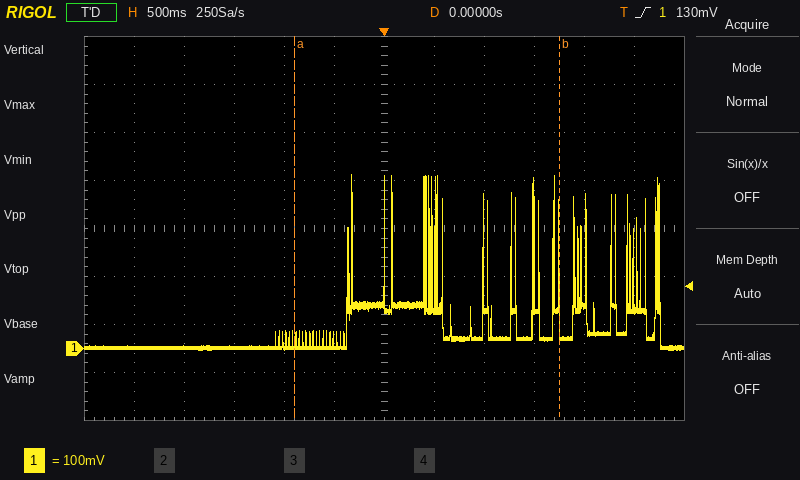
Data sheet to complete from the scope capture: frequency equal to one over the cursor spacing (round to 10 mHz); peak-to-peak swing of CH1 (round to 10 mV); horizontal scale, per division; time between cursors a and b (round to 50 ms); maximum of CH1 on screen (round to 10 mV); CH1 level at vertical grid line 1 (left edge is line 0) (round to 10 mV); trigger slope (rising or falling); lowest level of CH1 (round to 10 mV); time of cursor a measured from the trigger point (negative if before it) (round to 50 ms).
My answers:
380 mHz
360 mV
500 ms
2.65 s
360 mV
0 mV
rising
0 mV
-900 ms
